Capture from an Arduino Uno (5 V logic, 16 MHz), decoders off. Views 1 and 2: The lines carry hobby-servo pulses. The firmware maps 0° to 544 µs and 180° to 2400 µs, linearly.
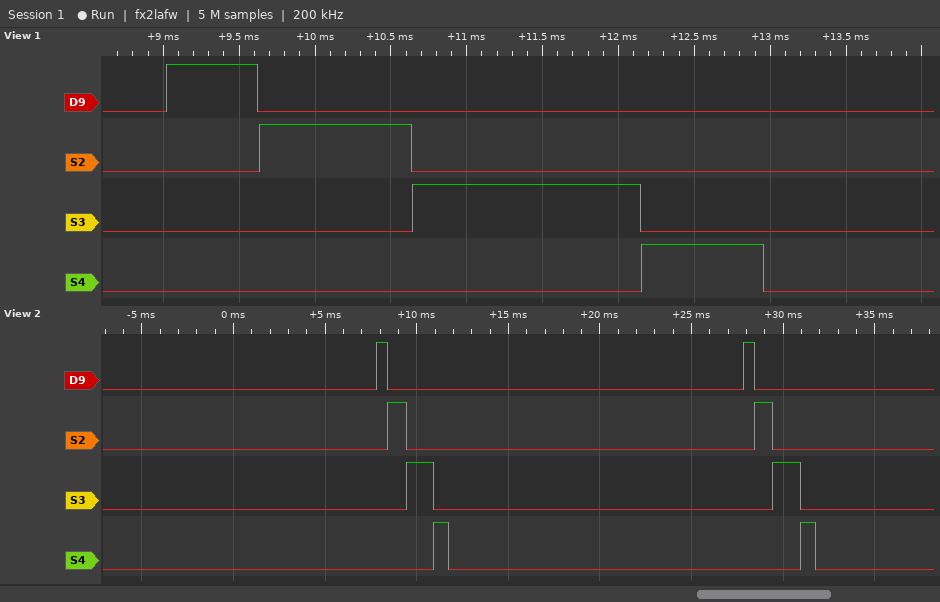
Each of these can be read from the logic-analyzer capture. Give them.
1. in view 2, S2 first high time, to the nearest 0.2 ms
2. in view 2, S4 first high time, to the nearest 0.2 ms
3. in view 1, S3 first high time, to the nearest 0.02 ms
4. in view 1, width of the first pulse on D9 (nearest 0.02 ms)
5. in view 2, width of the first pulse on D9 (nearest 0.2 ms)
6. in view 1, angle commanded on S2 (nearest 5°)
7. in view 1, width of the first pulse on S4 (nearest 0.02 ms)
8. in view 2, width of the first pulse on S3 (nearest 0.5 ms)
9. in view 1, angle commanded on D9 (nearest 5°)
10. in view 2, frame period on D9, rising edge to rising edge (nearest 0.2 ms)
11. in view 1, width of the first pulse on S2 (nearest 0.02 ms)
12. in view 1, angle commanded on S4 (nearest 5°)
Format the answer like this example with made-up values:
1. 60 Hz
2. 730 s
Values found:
1. 1.0 ms
2. 0.8 ms
3. 1.50 ms
4. 0.60 ms
5. 0.6 ms
6. 45°
7. 0.80 ms
8. 1.5 ms
9. 5°
10. 20.0 ms
11. 1.00 ms
12. 25°
